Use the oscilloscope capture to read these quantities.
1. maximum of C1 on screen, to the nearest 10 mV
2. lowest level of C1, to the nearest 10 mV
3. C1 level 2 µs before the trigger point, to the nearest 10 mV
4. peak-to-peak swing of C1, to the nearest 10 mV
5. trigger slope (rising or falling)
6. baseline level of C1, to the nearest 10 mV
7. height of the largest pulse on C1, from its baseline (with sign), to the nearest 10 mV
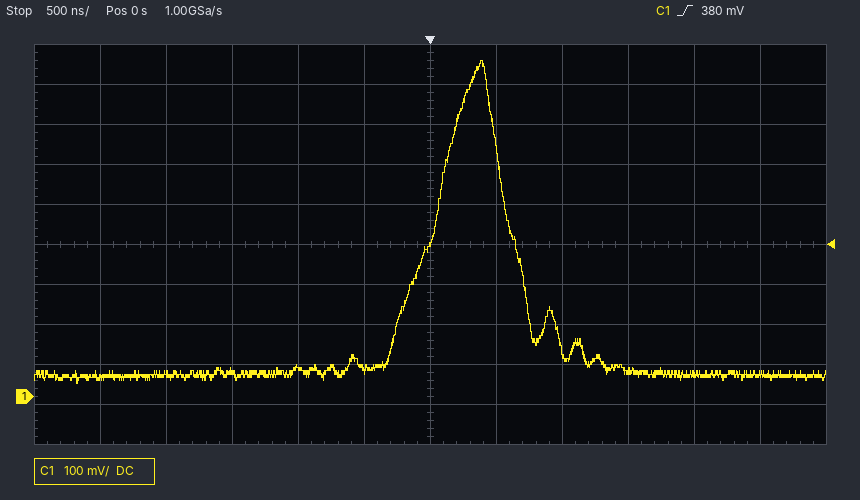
840 mV
30 mV
60 mV
810 mV
rising
60 mV
+780 mV
